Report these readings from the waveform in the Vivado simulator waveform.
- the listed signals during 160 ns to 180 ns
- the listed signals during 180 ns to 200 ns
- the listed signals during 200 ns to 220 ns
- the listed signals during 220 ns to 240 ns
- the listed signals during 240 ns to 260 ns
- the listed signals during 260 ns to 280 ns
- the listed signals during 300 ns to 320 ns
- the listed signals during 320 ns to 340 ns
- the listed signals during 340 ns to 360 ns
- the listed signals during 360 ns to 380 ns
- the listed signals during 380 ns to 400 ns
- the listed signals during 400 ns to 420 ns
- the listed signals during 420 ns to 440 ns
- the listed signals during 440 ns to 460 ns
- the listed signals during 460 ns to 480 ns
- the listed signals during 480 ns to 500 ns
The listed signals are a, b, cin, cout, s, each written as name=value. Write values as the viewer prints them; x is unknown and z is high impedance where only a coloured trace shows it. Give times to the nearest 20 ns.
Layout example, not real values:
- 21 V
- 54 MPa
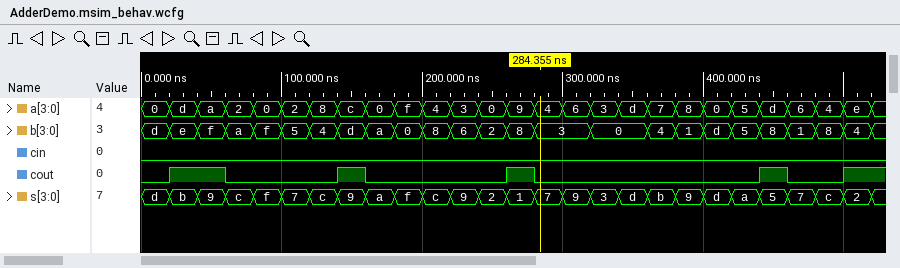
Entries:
- a=0, b=a, cin=0, cout=0, s=a
- a=f, b=0, cin=0, cout=0, s=f
- a=4, b=8, cin=0, cout=0, s=c
- a=3, b=6, cin=0, cout=0, s=9
- a=0, b=2, cin=0, cout=0, s=2
- a=9, b=8, cin=0, cout=1, s=1
- a=6, b=3, cin=0, cout=0, s=9
- a=3, b=0, cin=0, cout=0, s=3
- a=d, b=0, cin=0, cout=0, s=d
- a=7, b=4, cin=0, cout=0, s=b
- a=8, b=1, cin=0, cout=0, s=9
- a=0, b=d, cin=0, cout=0, s=d
- a=5, b=5, cin=0, cout=0, s=a
- a=d, b=8, cin=0, cout=1, s=5
- a=6, b=1, cin=0, cout=0, s=7
- a=4, b=8, cin=0, cout=0, s=c
